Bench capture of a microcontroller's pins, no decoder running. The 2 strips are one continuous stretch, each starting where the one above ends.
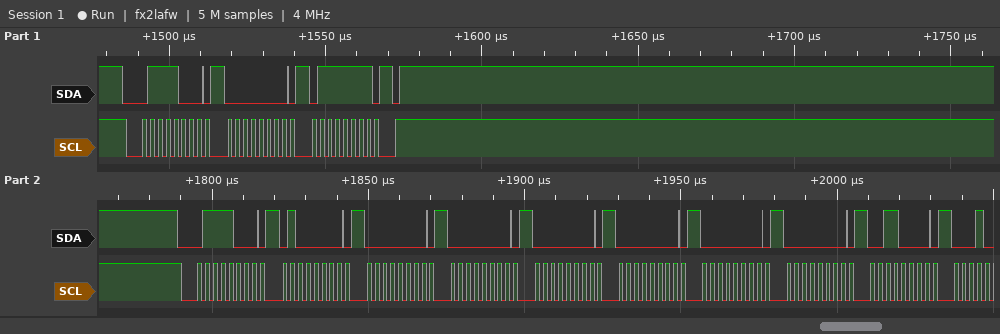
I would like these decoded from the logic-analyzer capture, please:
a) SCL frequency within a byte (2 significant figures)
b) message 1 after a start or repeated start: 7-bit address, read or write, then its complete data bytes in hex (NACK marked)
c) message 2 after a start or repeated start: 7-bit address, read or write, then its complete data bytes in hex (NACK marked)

400 kHz
0x3C write: 00 7F
0x3C write: 40 00 00 00 00 00 00 30
